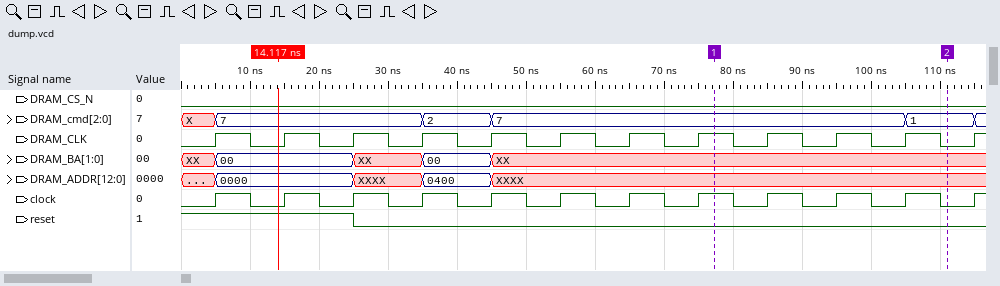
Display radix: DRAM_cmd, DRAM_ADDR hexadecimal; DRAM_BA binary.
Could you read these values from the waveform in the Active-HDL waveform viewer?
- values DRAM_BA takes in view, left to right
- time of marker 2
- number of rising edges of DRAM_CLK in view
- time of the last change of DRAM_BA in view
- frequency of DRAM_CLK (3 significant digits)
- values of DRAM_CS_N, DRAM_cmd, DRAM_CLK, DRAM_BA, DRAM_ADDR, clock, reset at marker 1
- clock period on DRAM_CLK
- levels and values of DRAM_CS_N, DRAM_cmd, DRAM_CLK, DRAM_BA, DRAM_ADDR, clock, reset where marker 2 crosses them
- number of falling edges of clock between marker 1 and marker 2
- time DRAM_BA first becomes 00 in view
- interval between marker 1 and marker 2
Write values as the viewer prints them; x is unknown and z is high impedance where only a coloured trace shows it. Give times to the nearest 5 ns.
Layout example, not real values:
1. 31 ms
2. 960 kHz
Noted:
1. XX, 00, XX, 00, XX
2. 110 ns
3. 12
4. 45 ns
5. 100 MHz
6. DRAM_CS_N=0, DRAM_cmd=7, DRAM_CLK=1, DRAM_BA=XX, DRAM_ADDR=XXXX, clock=1, reset=0
7. 10 ns
8. DRAM_CS_N=0, DRAM_cmd=1, DRAM_CLK=0, DRAM_BA=XX, DRAM_ADDR=XXXX, clock=0, reset=0
9. 4
10. 5 ns
11. 35 ns
